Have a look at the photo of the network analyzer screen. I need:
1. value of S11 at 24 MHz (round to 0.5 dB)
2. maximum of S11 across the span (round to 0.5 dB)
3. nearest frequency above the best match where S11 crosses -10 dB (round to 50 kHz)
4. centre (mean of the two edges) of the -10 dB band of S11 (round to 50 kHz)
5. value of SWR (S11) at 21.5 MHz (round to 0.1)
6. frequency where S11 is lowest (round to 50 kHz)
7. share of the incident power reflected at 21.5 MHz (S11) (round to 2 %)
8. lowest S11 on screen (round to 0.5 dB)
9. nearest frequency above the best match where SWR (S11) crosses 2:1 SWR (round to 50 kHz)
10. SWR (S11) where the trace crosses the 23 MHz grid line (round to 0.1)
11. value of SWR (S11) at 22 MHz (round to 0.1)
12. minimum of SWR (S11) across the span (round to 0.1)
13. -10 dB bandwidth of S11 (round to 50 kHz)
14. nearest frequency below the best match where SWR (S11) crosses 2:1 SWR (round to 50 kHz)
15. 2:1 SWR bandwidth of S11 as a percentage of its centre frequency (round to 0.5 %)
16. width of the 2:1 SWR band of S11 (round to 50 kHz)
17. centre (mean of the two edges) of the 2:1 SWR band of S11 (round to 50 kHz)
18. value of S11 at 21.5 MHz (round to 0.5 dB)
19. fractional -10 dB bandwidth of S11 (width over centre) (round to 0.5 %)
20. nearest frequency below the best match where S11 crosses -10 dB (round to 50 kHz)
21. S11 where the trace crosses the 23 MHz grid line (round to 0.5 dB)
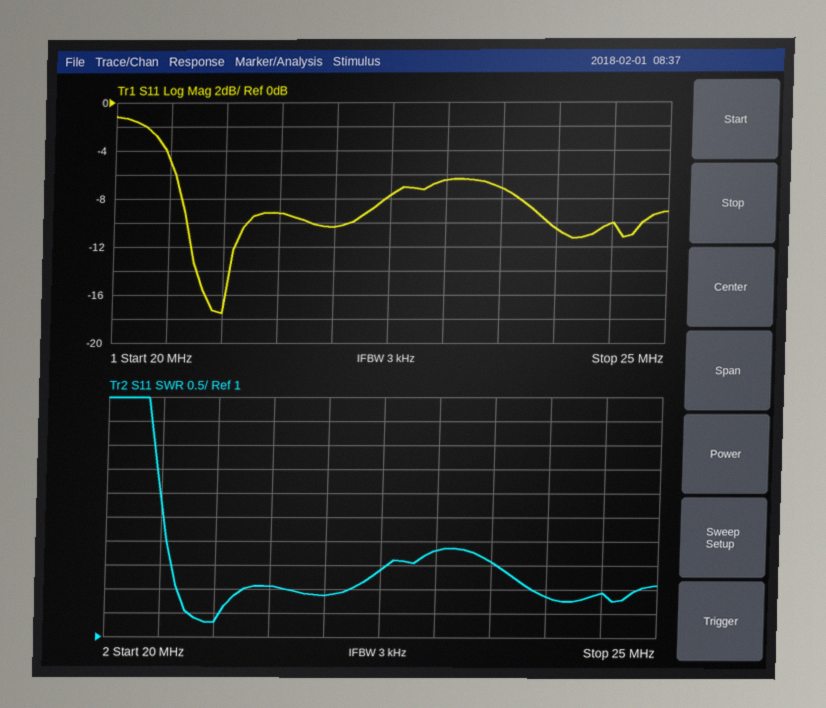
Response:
-10.5 dB
-1.0 dB
21.20 MHz
20.95 MHz
2.1
21.00 MHz
12 %
-17.5 dB
21.25 MHz
2.8
1.9
1.3
550 kHz
20.65 MHz
3.0 %
600 kHz
20.95 MHz
-9.0 dB
2.5 %
20.65 MHz
-6.5 dB
